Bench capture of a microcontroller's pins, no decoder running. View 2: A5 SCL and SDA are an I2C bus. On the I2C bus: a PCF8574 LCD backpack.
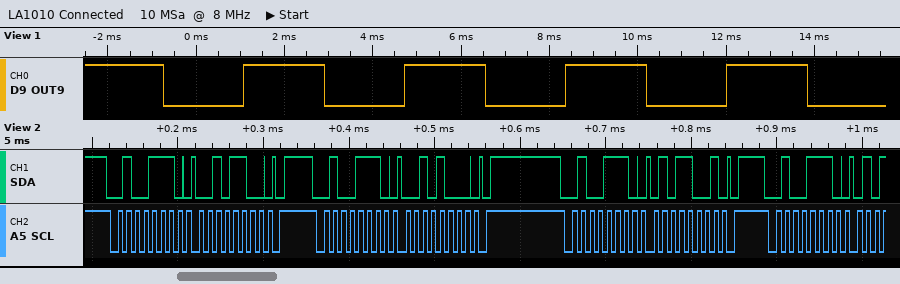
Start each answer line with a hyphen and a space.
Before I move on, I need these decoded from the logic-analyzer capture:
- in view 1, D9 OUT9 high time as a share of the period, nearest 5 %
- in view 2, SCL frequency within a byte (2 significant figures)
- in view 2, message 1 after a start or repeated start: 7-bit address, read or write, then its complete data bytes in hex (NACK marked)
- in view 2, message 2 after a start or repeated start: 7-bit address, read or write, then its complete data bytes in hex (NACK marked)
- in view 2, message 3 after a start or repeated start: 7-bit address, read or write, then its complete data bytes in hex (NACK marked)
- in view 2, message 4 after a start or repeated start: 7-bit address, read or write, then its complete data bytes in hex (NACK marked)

- 50 %
- 100 kHz
- 0x27 write: 2C
- 0x27 write: 28
- 0x27 write: 59
- 0x27 write
